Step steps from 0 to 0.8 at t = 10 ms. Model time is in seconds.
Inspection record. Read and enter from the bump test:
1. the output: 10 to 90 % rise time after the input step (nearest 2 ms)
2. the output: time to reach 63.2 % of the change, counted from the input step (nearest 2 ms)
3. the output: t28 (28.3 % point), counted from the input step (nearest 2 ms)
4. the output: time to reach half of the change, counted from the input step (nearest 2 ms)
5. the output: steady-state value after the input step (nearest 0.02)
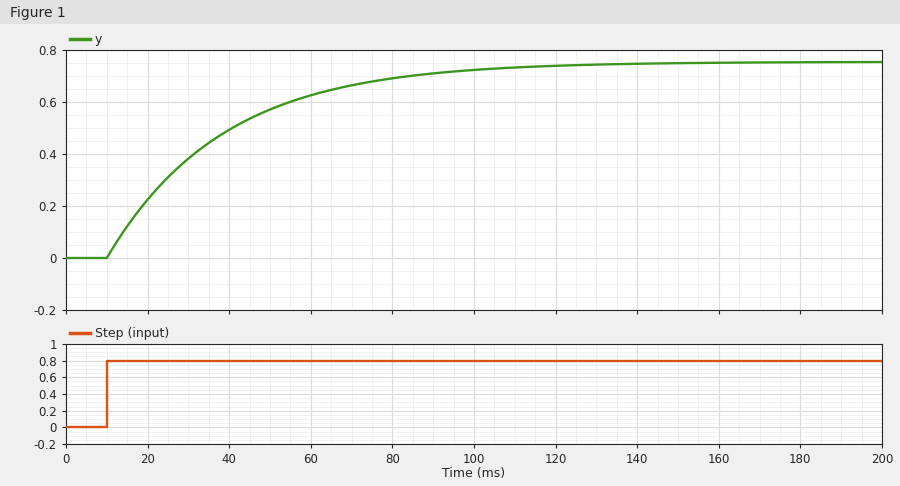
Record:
62 ms
28 ms
10 ms
20 ms
0.76
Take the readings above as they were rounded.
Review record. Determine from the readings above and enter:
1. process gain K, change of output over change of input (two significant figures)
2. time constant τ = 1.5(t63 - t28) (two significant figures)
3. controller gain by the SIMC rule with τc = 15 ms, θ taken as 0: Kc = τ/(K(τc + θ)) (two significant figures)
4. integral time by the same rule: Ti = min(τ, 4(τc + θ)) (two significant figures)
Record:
0.95
27 ms
1.9
27 ms
